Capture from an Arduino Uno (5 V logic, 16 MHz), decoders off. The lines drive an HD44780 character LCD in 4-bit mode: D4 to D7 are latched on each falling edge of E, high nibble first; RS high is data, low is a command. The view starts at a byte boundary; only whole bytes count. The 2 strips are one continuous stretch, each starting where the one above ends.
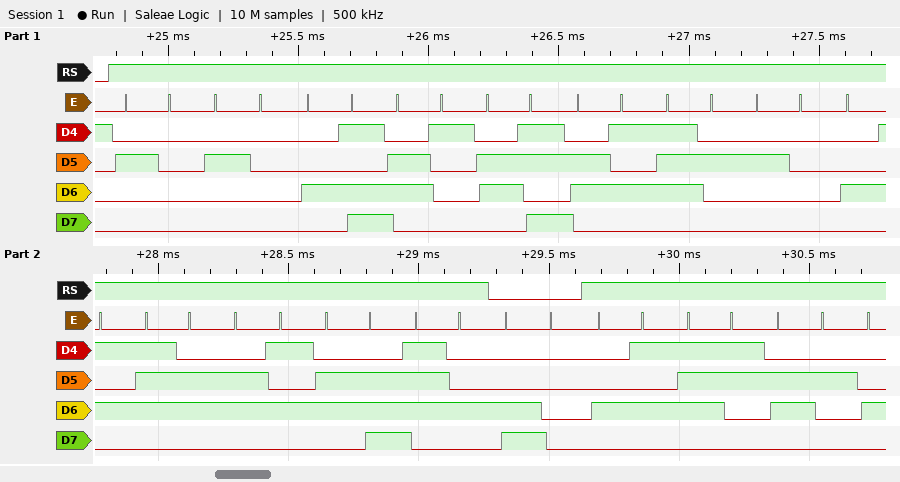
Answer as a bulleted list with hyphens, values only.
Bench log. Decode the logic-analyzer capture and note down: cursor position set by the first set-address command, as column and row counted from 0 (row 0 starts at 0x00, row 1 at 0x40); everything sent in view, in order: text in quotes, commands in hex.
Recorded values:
- column 0, row 1
- "  Maker Event" 0xC0 "Esb"
